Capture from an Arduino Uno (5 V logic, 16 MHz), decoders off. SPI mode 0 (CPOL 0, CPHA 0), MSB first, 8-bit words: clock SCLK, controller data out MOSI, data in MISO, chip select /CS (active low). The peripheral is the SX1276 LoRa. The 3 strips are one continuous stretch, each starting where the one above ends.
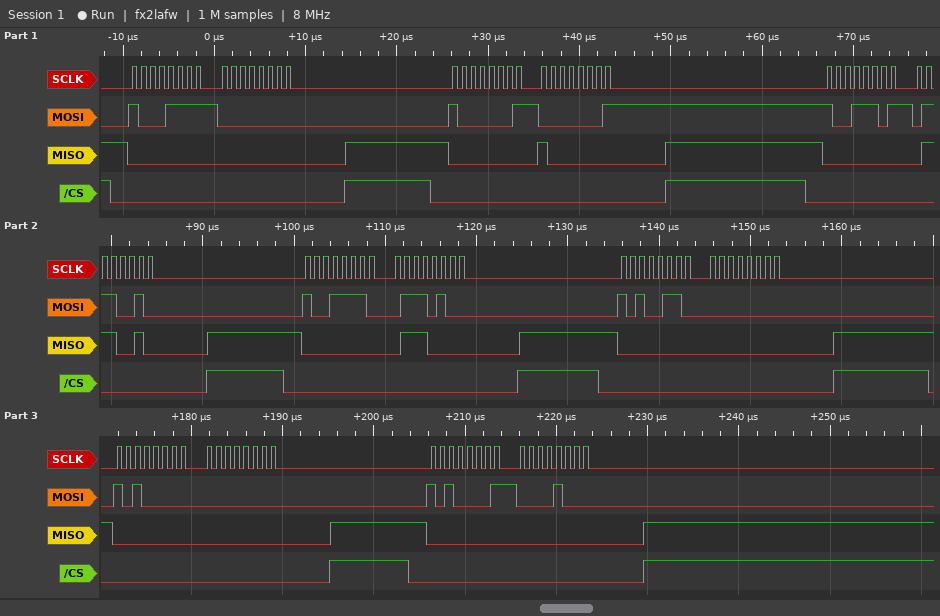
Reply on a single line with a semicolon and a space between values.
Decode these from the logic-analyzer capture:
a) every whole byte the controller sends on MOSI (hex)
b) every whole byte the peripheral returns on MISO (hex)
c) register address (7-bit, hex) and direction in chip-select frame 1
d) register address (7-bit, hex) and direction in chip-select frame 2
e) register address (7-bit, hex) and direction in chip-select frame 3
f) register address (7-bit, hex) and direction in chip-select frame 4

8F 00 81 01 9D 72 9E 74 A6 00 A0 00 A1 08; 00 00 00 80 00 72 00 70 00 00 00 00 00 00; 0x0F write; 0x01 write; 0x1D write; 0x1E write
